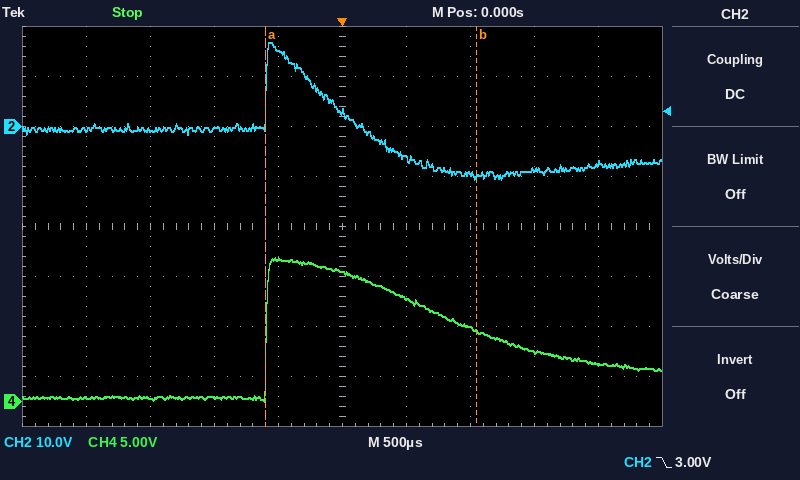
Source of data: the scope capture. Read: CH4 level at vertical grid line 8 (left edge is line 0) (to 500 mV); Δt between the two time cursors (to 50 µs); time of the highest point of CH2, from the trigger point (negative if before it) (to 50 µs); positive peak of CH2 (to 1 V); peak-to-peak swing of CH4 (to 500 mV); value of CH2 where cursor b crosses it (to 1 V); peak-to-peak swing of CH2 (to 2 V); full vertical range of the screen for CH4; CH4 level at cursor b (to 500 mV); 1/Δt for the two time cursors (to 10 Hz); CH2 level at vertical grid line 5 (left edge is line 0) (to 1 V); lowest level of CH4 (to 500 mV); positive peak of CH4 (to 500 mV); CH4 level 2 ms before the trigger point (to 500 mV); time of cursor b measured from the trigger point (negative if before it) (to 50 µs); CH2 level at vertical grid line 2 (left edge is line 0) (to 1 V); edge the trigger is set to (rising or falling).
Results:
5.0 V
1.65 ms
-550 µs
17 V
14.5 V
-10 V
28 V
40 V
7.0 V
610 Hz
3 V
0.0 V
14.5 V
500 mV
+1.05 ms
-1 V
falling
